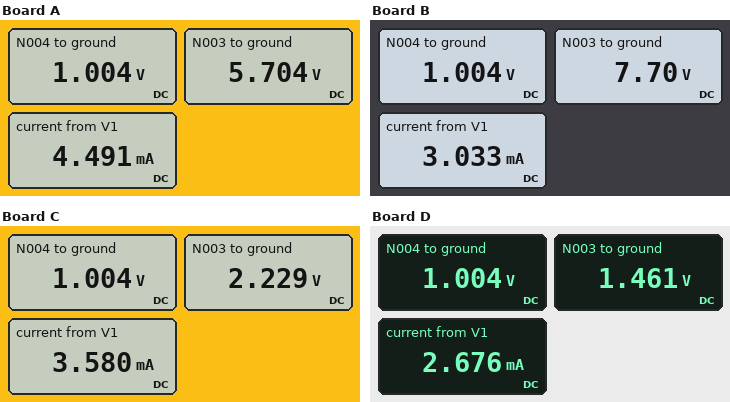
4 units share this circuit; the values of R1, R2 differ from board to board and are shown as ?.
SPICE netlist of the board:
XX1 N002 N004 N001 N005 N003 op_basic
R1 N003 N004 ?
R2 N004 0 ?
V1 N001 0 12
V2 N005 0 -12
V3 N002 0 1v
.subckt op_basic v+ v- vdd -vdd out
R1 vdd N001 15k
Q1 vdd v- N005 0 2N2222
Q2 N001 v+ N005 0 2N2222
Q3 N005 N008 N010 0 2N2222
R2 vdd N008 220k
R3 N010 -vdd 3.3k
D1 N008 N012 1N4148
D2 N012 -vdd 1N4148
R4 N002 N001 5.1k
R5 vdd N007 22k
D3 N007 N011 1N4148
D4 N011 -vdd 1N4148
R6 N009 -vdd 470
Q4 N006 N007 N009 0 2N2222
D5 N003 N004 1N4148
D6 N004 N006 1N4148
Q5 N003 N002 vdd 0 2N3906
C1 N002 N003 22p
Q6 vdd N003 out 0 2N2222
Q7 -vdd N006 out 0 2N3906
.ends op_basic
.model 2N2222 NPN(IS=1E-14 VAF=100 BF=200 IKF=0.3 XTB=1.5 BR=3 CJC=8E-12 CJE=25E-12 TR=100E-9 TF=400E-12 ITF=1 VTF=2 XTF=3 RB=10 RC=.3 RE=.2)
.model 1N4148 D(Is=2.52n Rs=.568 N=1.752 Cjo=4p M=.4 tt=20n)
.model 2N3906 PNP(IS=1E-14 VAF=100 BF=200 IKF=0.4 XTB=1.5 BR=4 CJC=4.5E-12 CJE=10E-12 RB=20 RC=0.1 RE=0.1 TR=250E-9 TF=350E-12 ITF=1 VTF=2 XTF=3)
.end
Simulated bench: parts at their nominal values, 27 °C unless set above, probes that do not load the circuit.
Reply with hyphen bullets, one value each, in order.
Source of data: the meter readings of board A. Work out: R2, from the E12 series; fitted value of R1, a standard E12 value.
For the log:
- 470 Ω
- 2.2 kΩ
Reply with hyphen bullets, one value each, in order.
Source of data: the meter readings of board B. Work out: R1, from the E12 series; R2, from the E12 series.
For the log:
- 10 kΩ
- 1.5 kΩ
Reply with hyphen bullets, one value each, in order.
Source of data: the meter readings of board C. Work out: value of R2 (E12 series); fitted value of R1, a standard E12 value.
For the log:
- 820 Ω
- 1 kΩ
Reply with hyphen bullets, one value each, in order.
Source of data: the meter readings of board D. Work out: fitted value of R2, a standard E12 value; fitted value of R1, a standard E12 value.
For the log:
- 3.3 kΩ
- 1.5 kΩ
